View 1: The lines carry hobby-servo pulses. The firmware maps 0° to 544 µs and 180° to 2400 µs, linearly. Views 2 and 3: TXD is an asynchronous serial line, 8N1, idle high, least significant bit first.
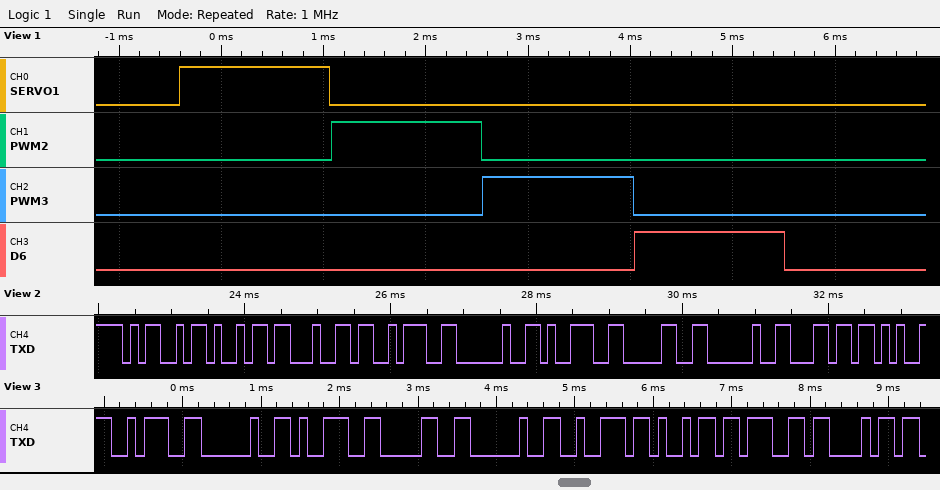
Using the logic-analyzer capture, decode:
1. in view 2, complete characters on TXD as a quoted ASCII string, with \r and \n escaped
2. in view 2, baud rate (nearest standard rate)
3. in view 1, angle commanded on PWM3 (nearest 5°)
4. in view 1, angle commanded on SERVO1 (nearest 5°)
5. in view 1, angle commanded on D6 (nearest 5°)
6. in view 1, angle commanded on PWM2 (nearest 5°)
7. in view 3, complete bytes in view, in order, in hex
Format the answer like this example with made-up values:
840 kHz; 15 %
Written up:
"Mid: 90 l"; 9600 baud; 90°; 90°; 90°; 90°; 0x3A 0x20 0x39 0x30 0x20 0x72 0x69 0x67 0x68
